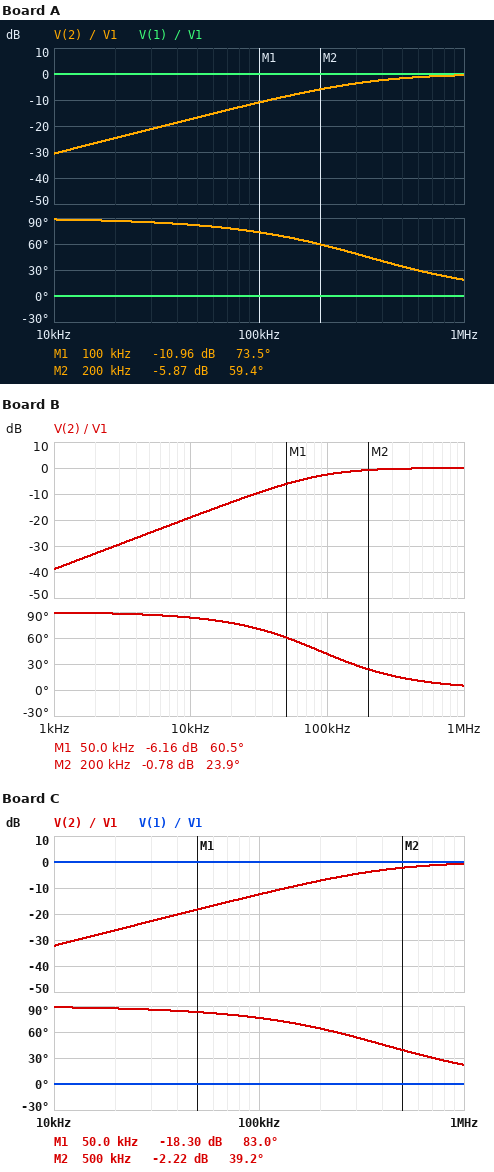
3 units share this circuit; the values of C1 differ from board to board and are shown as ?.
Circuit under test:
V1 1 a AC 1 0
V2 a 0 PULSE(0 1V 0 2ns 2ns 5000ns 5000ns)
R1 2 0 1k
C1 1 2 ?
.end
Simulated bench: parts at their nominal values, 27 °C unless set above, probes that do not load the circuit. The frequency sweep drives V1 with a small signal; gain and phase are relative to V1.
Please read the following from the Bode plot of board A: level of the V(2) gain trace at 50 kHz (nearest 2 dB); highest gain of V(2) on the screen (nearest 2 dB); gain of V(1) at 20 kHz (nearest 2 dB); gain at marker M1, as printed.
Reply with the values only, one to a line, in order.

-16 dB
0 dB
0 dB
-10.96 dB
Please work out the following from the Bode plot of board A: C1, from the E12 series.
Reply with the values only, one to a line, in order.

470 pF
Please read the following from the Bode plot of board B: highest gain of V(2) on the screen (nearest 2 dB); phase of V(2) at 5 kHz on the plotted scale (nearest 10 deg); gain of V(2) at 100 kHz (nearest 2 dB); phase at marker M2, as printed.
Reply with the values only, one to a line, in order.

0 dB
90 deg
-2 dB
23.9 deg
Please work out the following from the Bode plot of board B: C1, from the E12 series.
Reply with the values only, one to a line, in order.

1.8 nF
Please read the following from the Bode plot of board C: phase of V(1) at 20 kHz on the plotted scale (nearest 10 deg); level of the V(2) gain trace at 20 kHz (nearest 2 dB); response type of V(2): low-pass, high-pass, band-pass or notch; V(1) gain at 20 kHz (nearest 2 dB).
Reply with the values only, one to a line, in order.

0 deg
-26 dB
high-pass
0 dB
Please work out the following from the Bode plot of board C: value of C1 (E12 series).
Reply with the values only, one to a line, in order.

390 pF
